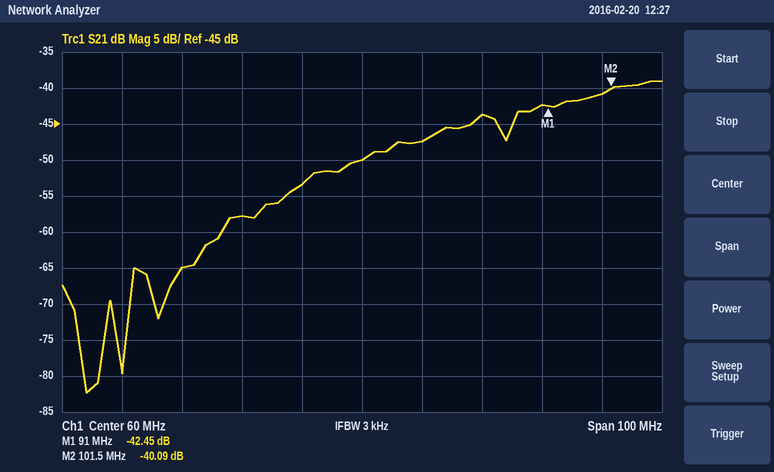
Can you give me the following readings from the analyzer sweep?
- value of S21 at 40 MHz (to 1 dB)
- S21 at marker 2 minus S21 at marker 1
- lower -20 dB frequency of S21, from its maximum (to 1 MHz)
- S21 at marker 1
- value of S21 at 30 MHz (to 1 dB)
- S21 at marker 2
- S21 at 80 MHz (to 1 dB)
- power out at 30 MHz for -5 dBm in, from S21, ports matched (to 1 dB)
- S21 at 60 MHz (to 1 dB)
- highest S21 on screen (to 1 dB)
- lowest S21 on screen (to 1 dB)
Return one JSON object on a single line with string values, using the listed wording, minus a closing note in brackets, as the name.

{"value of S21 at 40 MHz": "-58 dB", "S21 at marker 2 minus S21 at marker 1": "2.36 dB", "lower -20 dB frequency of S21, from its maximum": "37 MHz", "S21 at marker 1": "-42.45 dB", "value of S21 at 30 MHz": "-65 dB", "S21 at marker 2": "-40.09 dB", "S21 at 80 MHz": "-44 dB", "power out at 30 MHz for -5 dBm in, from S21, ports matched": "-70 dBm", "S21 at 60 MHz": "-50 dB", "highest S21 on screen": "-39 dB", "lowest S21 on screen": "-82 dB"}
